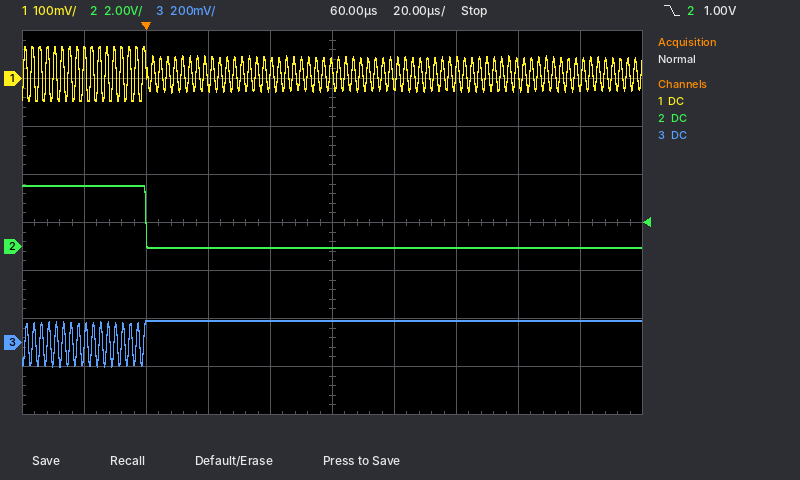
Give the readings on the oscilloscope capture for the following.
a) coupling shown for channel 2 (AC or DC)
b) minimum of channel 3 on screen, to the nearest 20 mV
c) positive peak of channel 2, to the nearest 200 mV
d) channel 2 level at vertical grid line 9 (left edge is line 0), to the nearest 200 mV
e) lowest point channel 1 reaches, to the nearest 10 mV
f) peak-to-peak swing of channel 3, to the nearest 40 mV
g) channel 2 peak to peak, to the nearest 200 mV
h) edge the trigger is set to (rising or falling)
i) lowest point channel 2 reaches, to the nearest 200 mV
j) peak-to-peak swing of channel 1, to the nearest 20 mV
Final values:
DC
-100 mV
2.6 V
0.0 V
-50 mV
200 mV
2.6 V
falling
0.0 V
120 mV
